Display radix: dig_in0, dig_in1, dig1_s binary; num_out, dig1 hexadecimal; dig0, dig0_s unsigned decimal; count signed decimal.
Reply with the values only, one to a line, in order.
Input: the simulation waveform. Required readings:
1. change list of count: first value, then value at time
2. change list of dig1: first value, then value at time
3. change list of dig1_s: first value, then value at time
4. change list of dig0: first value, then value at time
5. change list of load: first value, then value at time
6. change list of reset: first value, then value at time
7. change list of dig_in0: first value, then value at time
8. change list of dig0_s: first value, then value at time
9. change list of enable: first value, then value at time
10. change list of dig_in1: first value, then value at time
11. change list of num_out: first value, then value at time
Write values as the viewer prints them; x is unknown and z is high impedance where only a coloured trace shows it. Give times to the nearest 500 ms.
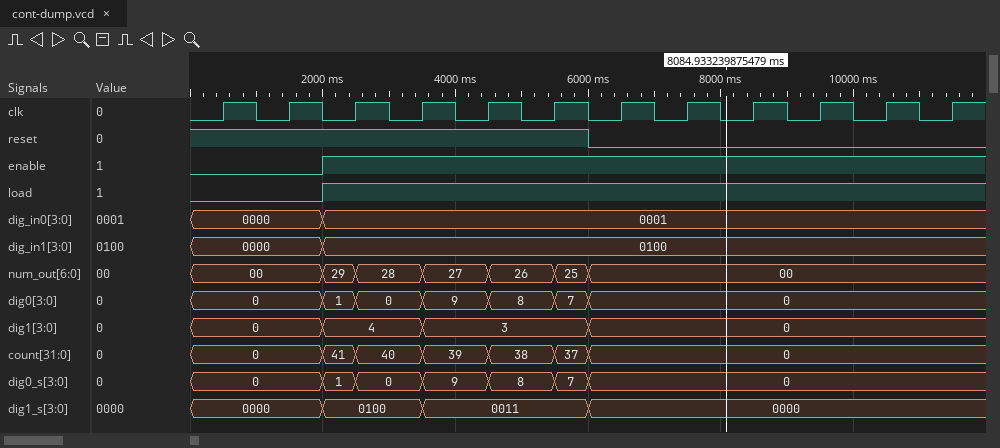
0, 41 at 2000 ms, 40 at 2500 ms, 39 at 3500 ms, 38 at 4500 ms, 37 at 5500 ms, 0 at 6000 ms
0, 4 at 2000 ms, 3 at 3500 ms, 0 at 6000 ms
0000, 0100 at 2000 ms, 0011 at 3500 ms, 0000 at 6000 ms
0, 1 at 2000 ms, 0 at 2500 ms, 9 at 3500 ms, 8 at 4500 ms, 7 at 5500 ms, 0 at 6000 ms
0, 1 at 2000 ms
1, 0 at 6000 ms
0000, 0001 at 2000 ms
0, 1 at 2000 ms, 0 at 2500 ms, 9 at 3500 ms, 8 at 4500 ms, 7 at 5500 ms, 0 at 6000 ms
0, 1 at 2000 ms
0000, 0100 at 2000 ms
00, 29 at 2000 ms, 28 at 2500 ms, 27 at 3500 ms, 26 at 4500 ms, 25 at 5500 ms, 00 at 6000 ms
